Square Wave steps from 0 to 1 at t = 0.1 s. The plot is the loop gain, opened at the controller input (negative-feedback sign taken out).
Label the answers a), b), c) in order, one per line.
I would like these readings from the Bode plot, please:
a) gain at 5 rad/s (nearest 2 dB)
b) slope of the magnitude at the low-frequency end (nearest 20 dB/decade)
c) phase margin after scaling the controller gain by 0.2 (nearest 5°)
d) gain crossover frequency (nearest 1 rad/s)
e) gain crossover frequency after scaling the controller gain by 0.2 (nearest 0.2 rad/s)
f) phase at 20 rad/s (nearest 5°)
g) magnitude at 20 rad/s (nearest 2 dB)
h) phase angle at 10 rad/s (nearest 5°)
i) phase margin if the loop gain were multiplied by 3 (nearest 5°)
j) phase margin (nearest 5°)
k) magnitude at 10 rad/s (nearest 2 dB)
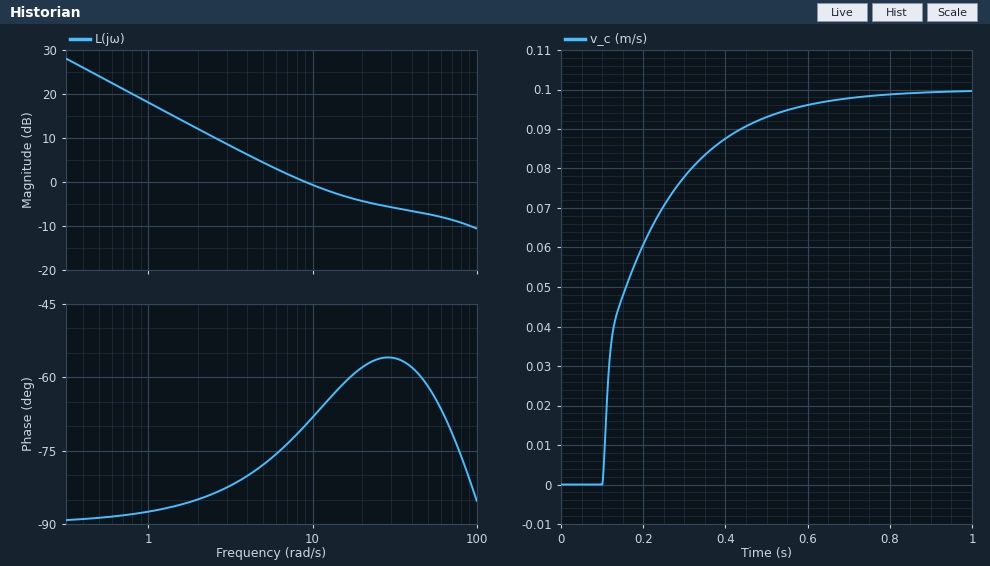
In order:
a) 4 dB
b) -20 dB/decade
c) 95°
d) 9 rad/s
e) 1.6 rad/s
f) -60°
g) -4 dB
h) -70°
i) 100°
j) 110°
k) 0 dB
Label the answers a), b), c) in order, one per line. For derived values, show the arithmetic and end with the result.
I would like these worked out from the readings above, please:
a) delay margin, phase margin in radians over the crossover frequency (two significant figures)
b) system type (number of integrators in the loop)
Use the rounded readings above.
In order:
a) 110 × π / 180 / 9 = 0.21 s
b) 1
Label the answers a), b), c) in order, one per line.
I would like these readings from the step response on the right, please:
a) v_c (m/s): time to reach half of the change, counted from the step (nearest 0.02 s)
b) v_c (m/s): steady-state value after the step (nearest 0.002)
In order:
a) 0.06 s
b) 0.100
